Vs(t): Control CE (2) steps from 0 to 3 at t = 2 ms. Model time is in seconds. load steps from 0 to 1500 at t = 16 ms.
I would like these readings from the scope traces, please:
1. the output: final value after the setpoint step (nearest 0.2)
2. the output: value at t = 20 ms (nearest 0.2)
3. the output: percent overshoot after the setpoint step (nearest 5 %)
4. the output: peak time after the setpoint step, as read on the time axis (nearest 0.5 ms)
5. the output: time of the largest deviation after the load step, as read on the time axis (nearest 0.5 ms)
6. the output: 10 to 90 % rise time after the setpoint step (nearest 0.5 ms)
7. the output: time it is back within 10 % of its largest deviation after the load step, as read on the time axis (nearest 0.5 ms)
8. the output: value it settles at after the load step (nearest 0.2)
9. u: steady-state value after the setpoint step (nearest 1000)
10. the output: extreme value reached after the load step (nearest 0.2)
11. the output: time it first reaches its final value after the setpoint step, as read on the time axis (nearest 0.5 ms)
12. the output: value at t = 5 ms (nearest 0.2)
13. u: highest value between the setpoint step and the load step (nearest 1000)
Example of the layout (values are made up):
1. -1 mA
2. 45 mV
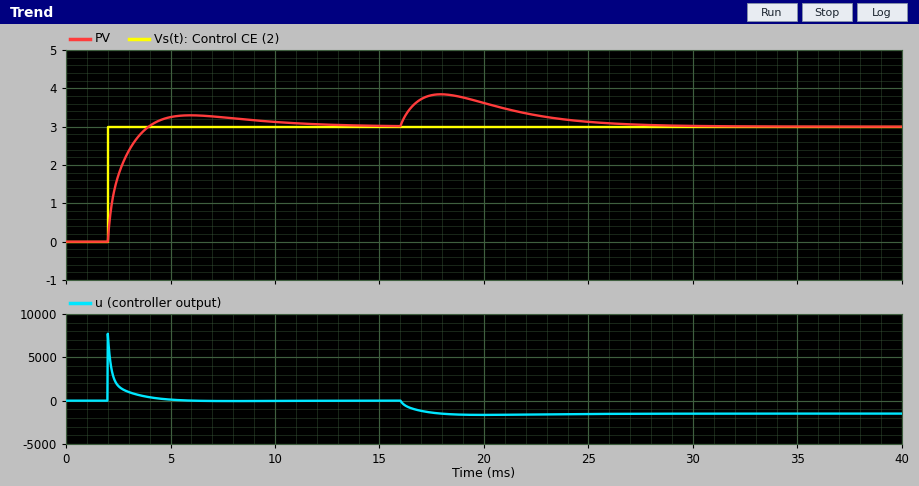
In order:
1. 3.0
2. 3.6
3. 10 %
4. 6.0 ms
5. 18.0 ms
6. 1.5 ms
7. 26.0 ms
8. 3.0
9. 0
10. 3.8
11. 4.0 ms
12. 3.2
13. 8000
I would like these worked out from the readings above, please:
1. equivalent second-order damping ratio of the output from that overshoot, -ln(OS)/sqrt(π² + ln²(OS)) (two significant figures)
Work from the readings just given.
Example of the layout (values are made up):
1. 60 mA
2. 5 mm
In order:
1. 0.59
